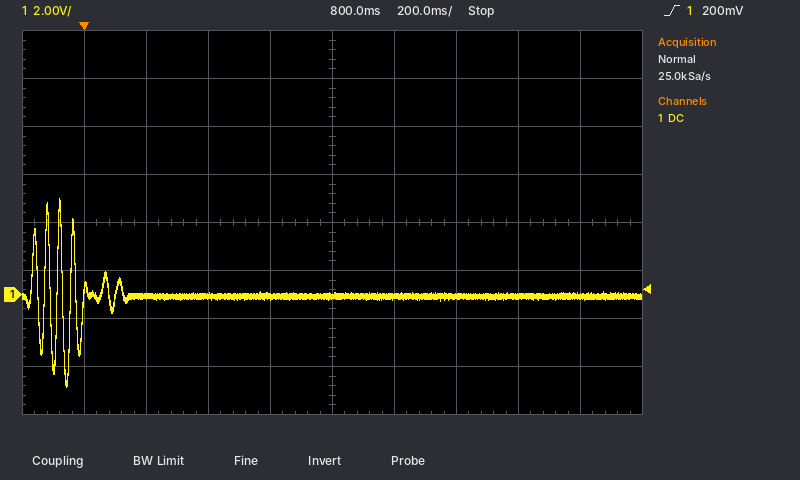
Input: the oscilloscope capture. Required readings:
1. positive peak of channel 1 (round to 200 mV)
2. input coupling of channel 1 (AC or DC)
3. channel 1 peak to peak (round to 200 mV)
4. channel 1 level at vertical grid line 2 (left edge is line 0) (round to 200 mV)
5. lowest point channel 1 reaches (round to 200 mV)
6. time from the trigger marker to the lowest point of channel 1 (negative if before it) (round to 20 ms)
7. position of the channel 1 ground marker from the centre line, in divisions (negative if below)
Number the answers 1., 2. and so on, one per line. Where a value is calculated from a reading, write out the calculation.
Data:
1. 4.0 V
2. DC
3. 4.0 V − (-3.8 V) = 7.8 V
4. 0.0 V
5. -3.8 V
6. -60 ms
7. -1.5 div
